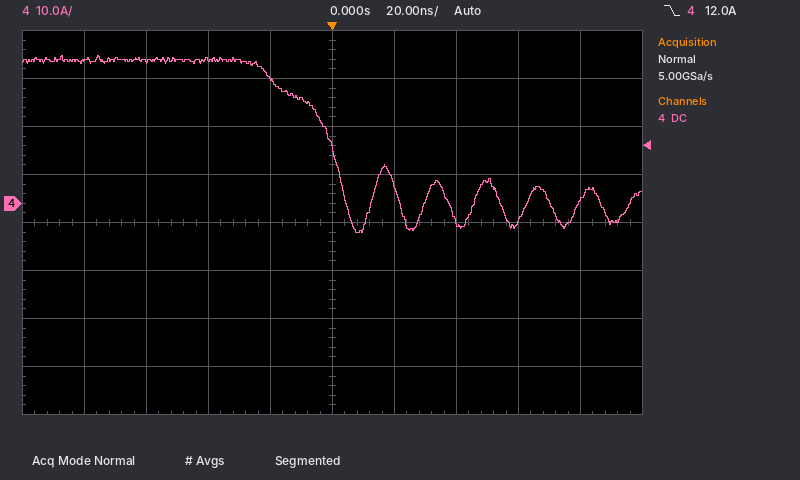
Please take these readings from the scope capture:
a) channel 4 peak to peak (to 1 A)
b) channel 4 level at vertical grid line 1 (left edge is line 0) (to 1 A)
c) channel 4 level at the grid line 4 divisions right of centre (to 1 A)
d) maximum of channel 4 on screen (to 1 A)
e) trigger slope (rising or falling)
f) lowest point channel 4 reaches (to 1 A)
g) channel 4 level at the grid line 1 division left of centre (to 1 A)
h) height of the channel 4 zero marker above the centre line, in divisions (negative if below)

37 A
30 A
0 A
31 A
falling
-6 A
26 A
+0.4 div
